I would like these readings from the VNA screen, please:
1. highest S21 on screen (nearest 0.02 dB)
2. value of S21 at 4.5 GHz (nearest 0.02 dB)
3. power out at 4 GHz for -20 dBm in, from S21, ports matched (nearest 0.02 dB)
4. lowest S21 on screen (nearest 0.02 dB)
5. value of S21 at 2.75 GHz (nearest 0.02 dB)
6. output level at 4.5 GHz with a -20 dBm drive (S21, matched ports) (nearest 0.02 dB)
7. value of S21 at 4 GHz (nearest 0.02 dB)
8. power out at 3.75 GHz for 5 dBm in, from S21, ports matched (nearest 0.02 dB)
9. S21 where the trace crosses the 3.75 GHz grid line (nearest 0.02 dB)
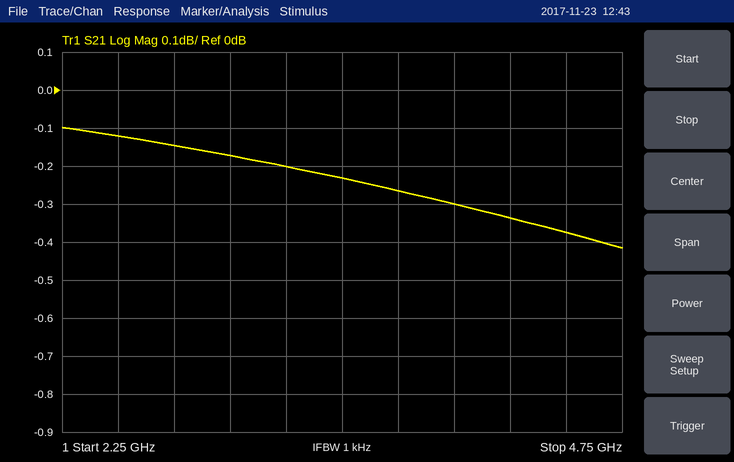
-0.10 dB
-0.38 dB
-20.30 dBm
-0.42 dB
-0.14 dB
-20.38 dBm
-0.30 dB
4.74 dBm
-0.26 dB
